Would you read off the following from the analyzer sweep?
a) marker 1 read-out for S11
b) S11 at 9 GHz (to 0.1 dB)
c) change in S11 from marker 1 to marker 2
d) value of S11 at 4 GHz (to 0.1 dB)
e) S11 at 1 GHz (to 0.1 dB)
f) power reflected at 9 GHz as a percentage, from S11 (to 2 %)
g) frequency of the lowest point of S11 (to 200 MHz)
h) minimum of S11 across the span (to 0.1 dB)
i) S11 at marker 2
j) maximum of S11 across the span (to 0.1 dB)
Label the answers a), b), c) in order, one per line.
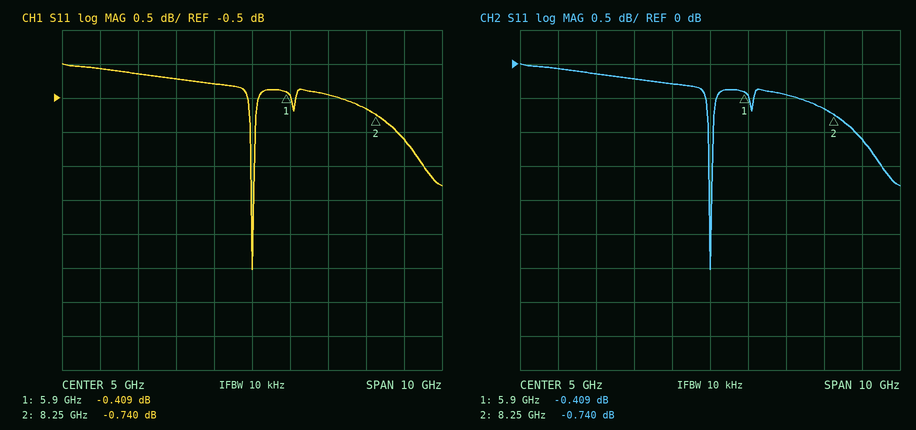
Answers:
a) -0.409 dB
b) -1.1 dB
c) -0.331 dB
d) -0.3 dB
e) -0.1 dB
f) 78 %
g) 5.0 GHz
h) -3.0 dB
i) -0.740 dB
j) 0.0 dB
